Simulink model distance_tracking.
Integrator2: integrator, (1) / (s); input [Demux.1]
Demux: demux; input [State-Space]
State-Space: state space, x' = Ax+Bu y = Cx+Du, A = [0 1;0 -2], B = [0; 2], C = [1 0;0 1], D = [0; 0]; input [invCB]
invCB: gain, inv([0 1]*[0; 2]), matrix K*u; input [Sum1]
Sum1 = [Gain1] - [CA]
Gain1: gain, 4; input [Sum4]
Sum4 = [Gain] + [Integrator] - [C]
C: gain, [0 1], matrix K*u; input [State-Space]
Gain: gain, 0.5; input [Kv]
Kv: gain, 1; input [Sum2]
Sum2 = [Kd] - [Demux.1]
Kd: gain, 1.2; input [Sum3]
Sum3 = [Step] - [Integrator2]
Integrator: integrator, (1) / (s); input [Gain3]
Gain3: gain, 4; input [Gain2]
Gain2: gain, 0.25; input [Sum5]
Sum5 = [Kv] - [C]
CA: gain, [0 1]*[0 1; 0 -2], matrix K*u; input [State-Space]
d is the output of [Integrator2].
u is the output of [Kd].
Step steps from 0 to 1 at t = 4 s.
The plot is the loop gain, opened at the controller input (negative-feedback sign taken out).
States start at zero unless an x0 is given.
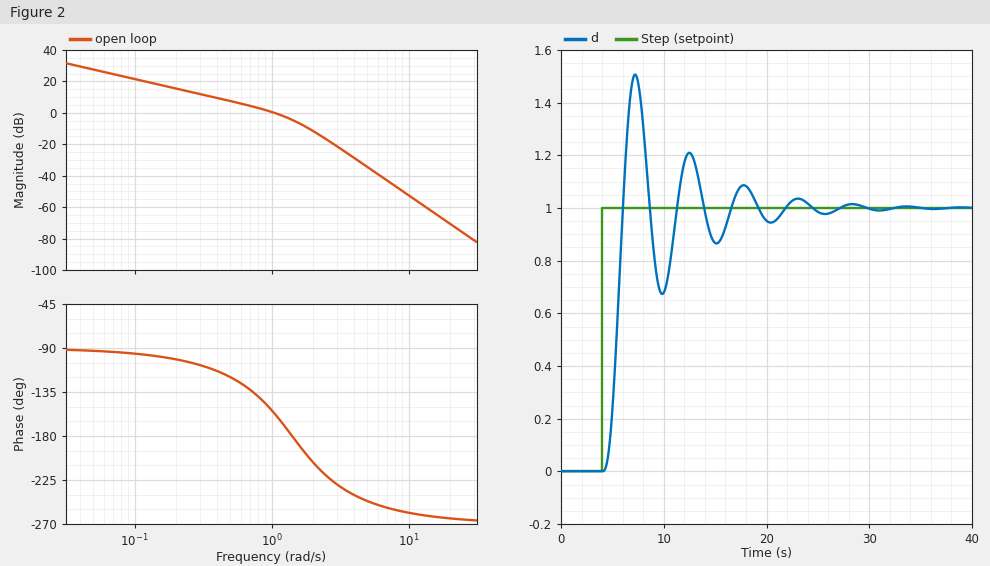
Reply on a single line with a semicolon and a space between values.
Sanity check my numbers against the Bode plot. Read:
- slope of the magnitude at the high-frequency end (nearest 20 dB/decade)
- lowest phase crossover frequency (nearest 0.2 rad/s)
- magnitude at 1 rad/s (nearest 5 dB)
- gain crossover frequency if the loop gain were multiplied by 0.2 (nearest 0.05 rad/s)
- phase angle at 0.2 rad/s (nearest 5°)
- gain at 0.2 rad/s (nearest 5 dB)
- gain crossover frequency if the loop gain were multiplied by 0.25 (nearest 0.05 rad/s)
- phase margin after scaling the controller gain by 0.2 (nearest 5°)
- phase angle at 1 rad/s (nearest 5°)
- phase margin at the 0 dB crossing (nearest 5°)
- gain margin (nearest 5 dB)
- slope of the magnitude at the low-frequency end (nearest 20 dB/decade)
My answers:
-60 dB/decade; 1.4 rad/s; 0 dB; 0.25 rad/s; -100°; 15 dB; 0.30 rad/s; 75°; -155°; 25°; 5 dB; -20 dB/decade
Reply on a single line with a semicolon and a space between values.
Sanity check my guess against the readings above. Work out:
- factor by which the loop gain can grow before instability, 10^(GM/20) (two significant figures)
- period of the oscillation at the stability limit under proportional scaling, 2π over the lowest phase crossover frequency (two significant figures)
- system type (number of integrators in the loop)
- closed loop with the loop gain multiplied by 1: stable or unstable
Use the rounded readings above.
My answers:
1.8; 4.5 s; 1; stable
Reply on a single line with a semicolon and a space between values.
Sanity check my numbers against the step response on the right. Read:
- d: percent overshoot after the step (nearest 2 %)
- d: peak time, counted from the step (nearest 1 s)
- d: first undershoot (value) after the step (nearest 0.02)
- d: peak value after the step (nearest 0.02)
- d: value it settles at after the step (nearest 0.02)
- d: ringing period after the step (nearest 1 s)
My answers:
50 %; 3 s; 0.68; 1.50; 1.00; 5 s
